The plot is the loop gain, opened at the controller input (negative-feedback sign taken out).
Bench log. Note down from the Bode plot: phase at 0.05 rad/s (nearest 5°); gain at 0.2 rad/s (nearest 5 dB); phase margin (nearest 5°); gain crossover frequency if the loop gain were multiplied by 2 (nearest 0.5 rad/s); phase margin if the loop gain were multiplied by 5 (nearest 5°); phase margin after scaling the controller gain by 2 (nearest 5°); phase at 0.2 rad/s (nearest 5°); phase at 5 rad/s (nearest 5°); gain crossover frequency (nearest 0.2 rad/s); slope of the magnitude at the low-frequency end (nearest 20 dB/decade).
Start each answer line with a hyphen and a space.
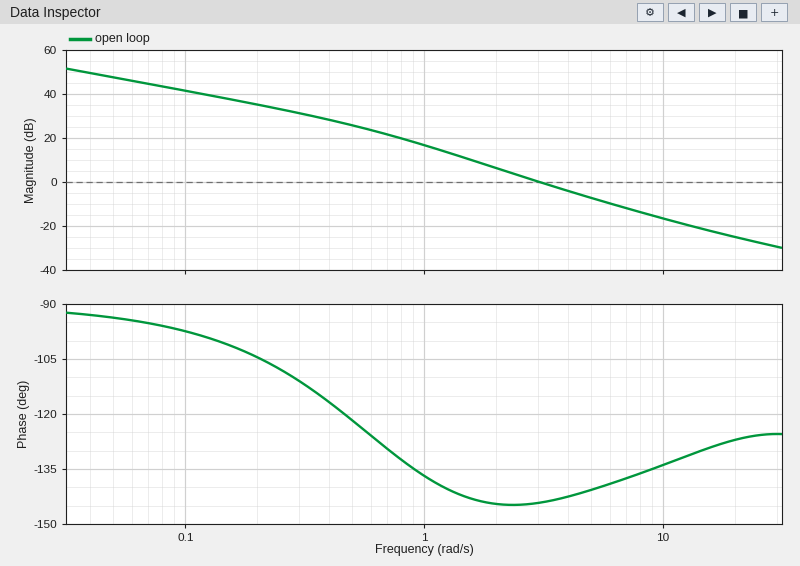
- -95°
- 35 dB
- 35°
- 4.5 rad/s
- 45°
- 40°
- -105°
- -140°
- 3.0 rad/s
- -20 dB/decade
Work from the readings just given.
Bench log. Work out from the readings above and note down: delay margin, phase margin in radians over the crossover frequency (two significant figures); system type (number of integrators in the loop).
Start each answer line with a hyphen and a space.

- 0.20 s
- 1
